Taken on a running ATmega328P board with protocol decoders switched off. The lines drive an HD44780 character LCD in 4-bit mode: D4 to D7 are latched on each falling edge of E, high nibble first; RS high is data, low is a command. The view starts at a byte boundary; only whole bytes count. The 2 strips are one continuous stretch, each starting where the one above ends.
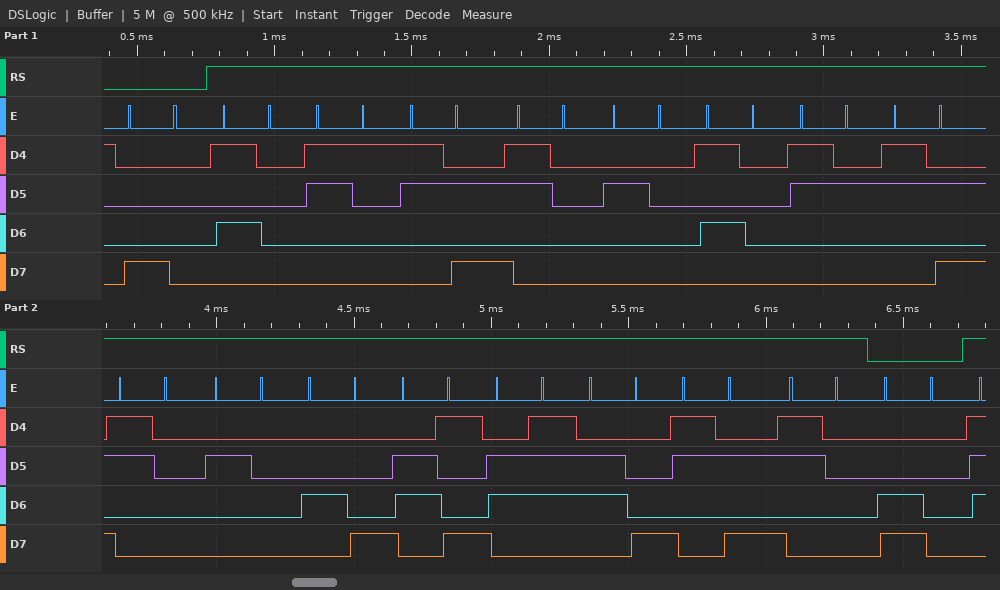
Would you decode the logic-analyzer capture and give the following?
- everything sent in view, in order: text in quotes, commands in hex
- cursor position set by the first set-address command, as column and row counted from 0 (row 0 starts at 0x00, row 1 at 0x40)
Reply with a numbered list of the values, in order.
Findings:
1. 0x80 "P1:0 P2:0 High:0" 0xC0
2. column 0, row 0
